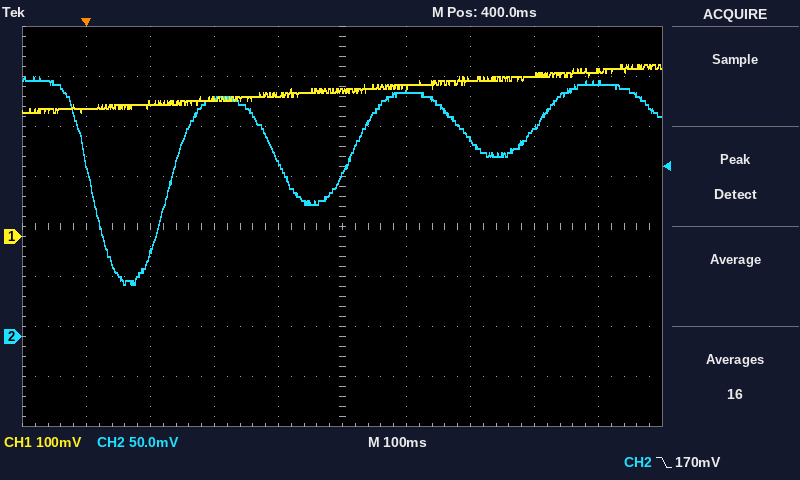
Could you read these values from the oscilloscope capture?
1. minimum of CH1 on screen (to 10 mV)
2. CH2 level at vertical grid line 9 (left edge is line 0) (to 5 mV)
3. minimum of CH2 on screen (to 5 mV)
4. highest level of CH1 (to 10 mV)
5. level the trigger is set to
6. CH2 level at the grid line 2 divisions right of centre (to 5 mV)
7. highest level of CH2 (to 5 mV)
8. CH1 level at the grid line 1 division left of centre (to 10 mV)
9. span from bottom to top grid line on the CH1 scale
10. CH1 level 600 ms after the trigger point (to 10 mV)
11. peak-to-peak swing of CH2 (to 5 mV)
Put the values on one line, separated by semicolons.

250 mV; 255 mV; 50 mV; 340 mV; 170 mV; 195 mV; 260 mV; 280 mV; 800 mV; 320 mV; 210 mV
